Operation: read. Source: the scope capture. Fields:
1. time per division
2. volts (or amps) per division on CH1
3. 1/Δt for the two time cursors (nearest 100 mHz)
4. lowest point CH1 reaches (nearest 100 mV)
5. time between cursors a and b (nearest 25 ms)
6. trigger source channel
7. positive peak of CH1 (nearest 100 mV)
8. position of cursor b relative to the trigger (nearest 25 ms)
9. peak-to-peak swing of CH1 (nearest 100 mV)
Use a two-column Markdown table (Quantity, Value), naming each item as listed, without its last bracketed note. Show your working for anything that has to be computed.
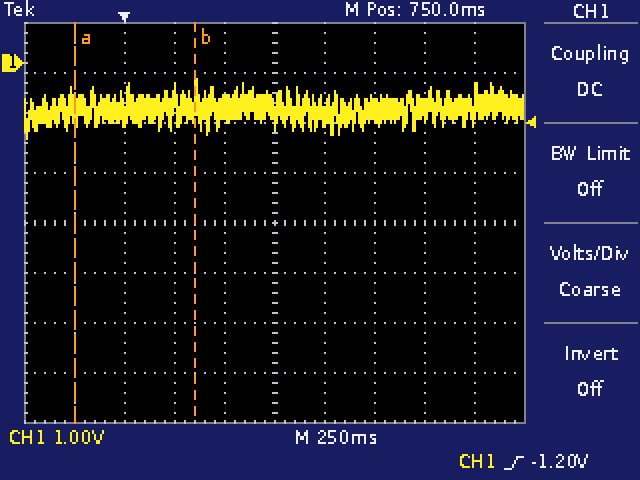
| Quantity | Value |
|---|---|
| time per division | 250 ms |
| volts (or amps) per division on CH1 | 1 V |
| 1/Δt for the two time cursors | 1 / 600 ms ≈ 1.7 Hz |
| lowest point CH1 reaches | -1.5 V |
| time between cursors a and b | 600 ms |
| trigger source channel | CH1 |
| positive peak of CH1 | -300 mV |
| position of cursor b relative to the trigger | +350 ms |
| peak-to-peak swing of CH1 | -300 mV − (-1.5 V) = 1.2 V |
